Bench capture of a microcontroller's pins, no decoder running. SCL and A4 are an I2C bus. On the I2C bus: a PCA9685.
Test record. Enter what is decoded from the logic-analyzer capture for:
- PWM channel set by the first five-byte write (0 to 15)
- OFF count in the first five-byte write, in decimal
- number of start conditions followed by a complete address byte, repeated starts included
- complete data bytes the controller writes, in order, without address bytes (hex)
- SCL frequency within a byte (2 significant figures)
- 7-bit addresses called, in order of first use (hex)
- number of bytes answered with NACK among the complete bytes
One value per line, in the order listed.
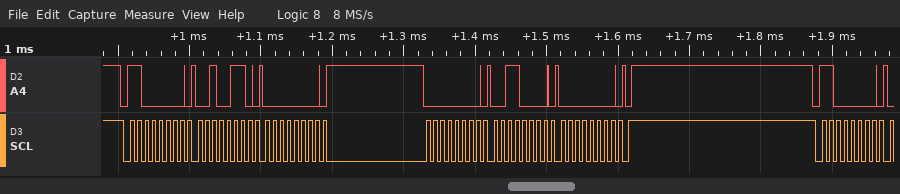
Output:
8
48
2
26 00 00 30 00
100 kHz
0x60
0
